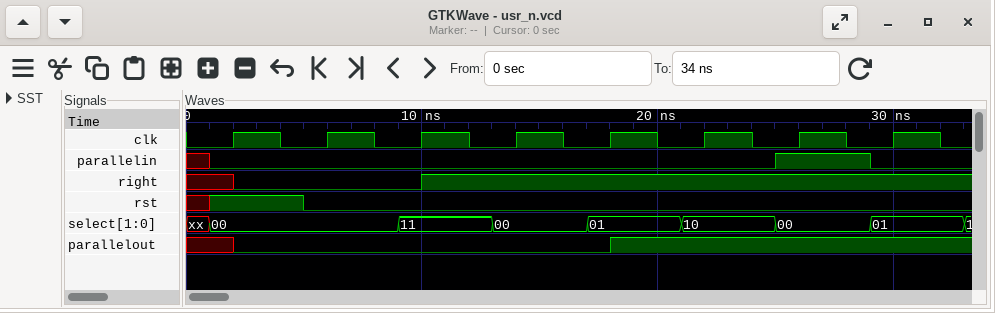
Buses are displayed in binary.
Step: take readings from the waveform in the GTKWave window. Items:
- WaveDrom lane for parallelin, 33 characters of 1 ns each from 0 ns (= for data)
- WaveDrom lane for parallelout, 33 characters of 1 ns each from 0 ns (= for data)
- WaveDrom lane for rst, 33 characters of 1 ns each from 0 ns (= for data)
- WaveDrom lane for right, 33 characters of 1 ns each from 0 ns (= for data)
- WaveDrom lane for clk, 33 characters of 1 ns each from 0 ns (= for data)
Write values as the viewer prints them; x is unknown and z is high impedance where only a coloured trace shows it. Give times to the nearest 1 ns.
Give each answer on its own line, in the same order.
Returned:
{name: 'parallelin', wave: 'x0.......................1...0...'}
{name: 'parallelout', wave: 'x.0...............1..............'}
{name: 'rst', wave: 'x1...0...........................'}
{name: 'right', wave: 'x.0.......1......................'}
{name: 'clk', wave: '0.1.0.1.0.1.0.1.0.1.0.1.0.1.0.1.0'}
